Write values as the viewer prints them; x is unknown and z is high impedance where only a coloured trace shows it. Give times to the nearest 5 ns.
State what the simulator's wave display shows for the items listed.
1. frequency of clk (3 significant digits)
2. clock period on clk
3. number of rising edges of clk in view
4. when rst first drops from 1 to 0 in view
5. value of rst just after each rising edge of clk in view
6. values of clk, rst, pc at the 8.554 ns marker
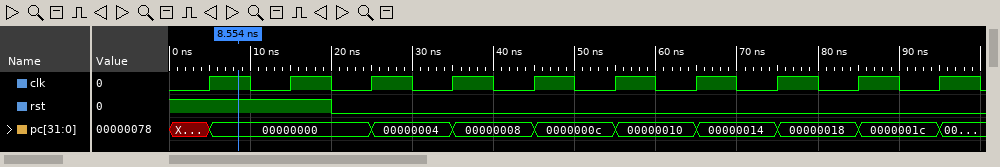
100 MHz
10 ns
10
20 ns
1 1 0 0 0 0 0 0 0 0
clk=1, rst=1, pc=00000000
